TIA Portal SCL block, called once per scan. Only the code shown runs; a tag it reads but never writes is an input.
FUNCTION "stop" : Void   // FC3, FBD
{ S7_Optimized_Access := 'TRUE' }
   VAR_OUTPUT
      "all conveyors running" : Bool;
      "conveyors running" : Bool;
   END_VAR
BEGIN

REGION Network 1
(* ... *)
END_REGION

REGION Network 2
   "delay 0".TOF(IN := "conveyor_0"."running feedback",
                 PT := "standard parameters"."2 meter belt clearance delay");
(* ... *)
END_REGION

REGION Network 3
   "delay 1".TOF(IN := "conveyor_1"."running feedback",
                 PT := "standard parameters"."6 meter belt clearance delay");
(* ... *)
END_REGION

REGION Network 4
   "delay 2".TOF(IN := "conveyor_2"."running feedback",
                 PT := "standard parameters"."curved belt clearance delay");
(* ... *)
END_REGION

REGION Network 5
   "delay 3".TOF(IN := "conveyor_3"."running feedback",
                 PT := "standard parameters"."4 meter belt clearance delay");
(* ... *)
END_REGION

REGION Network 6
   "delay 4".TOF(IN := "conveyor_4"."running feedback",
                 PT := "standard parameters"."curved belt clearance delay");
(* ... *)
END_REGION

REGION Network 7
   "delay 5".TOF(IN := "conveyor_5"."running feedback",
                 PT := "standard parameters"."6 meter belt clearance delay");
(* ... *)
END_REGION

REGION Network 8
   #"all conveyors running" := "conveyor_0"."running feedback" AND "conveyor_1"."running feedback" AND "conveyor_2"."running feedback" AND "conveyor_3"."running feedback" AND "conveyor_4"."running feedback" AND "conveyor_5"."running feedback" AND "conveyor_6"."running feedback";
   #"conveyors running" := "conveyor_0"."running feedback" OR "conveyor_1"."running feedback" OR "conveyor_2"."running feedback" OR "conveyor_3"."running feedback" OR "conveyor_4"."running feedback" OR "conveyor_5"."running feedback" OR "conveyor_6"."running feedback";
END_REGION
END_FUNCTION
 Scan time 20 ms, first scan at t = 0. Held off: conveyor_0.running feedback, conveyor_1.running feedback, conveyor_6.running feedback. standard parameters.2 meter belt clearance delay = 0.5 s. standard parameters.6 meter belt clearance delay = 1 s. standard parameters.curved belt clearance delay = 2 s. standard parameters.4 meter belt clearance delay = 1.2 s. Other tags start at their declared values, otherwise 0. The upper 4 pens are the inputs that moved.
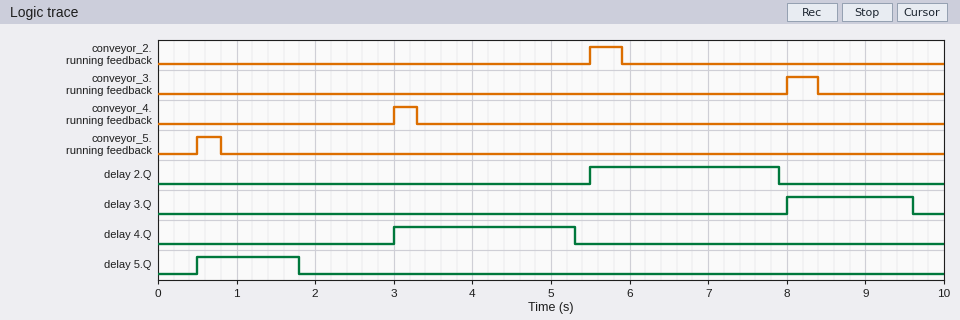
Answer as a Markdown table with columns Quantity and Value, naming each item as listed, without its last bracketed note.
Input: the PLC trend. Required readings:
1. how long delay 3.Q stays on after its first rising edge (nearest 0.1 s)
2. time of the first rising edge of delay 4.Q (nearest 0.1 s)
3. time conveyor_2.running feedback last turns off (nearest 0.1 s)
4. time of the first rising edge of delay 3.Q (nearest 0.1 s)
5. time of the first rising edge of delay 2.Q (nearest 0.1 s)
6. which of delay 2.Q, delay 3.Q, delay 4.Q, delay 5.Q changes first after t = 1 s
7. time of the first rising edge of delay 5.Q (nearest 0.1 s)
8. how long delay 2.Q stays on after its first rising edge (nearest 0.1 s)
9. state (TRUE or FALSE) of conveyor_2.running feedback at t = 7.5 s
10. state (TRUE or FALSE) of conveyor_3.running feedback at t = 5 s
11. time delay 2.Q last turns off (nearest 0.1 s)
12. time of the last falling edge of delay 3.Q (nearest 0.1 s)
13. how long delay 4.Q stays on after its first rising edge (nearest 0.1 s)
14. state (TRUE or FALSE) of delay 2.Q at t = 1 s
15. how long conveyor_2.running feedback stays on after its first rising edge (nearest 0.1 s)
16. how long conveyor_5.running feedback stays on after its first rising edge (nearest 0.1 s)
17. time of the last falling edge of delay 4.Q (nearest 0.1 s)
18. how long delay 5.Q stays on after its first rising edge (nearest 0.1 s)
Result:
| Quantity | Value |
|---|---|
| how long delay 3.Q stays on after its first rising edge | 1.6 s |
| time of the first rising edge of delay 4.Q | 3.0 s |
| time conveyor_2.running feedback last turns off | 5.9 s |
| time of the first rising edge of delay 3.Q | 8.0 s |
| time of the first rising edge of delay 2.Q | 5.5 s |
| which of delay 2.Q, delay 3.Q, delay 4.Q, delay 5.Q changes first after t = 1 s | delay 5.Q |
| time of the first rising edge of delay 5.Q | 0.5 s |
| how long delay 2.Q stays on after its first rising edge | 2.4 s |
| state (TRUE or FALSE) of conveyor_2.running feedback at t = 7.5 s | FALSE |
| state (TRUE or FALSE) of conveyor_3.running feedback at t = 5 s | FALSE |
| time delay 2.Q last turns off | 7.9 s |
| time of the last falling edge of delay 3.Q | 9.6 s |
| how long delay 4.Q stays on after its first rising edge | 2.3 s |
| state (TRUE or FALSE) of delay 2.Q at t = 1 s | FALSE |
| how long conveyor_2.running feedback stays on after its first rising edge | 0.4 s |
| how long conveyor_5.running feedback stays on after its first rising edge | 0.3 s |
| time of the last falling edge of delay 4.Q | 5.3 s |
| how long delay 5.Q stays on after its first rising edge | 1.3 s |
